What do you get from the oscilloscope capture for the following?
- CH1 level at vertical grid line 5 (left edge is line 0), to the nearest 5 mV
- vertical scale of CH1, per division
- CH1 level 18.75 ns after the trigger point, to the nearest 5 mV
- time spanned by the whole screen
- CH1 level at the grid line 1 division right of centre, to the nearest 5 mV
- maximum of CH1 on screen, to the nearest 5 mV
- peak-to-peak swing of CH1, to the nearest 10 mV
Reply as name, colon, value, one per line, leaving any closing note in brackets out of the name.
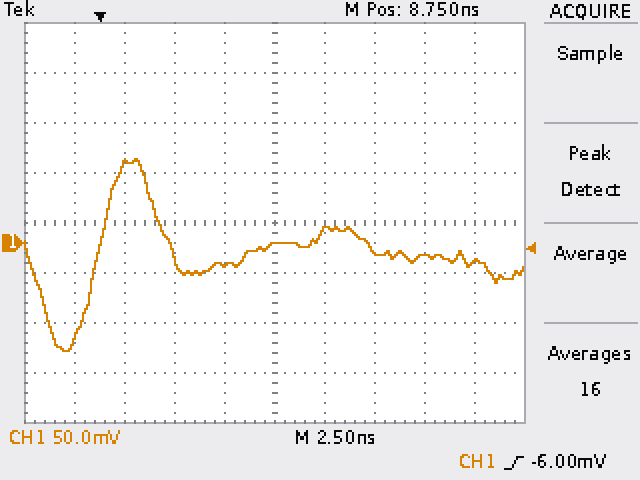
CH1 level at vertical grid line 5 (left edge is line 0), to the nearest 5 mV: 0 mV
vertical scale of CH1, per division: 50 mV
CH1 level 18.75 ns after the trigger point, to the nearest 5 mV: -20 mV
time spanned by the whole screen: 25 ns
CH1 level at the grid line 1 division right of centre, to the nearest 5 mV: 10 mV
maximum of CH1 on screen, to the nearest 5 mV: 85 mV
peak-to-peak swing of CH1, to the nearest 10 mV: 190 mV
